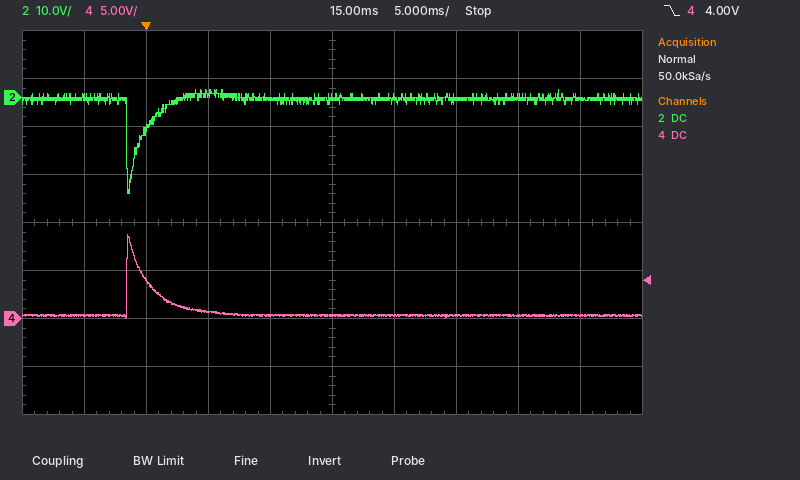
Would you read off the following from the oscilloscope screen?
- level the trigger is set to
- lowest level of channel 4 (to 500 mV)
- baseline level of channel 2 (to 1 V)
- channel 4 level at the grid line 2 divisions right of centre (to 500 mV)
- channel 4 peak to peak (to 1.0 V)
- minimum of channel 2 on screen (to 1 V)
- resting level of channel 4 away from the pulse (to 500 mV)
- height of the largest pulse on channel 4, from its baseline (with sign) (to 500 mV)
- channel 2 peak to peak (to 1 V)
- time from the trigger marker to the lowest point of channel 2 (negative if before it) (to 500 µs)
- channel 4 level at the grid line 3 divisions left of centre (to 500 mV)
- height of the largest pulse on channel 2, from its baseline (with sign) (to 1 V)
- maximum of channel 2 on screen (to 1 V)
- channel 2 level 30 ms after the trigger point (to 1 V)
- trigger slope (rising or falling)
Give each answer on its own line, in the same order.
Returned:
4.00 V
0.0 V
0 V
500 mV
9.0 V
-20 V
500 mV
+8.5 V
22 V
-1.5 ms
4.0 V
-20 V
2 V
0 V
falling
